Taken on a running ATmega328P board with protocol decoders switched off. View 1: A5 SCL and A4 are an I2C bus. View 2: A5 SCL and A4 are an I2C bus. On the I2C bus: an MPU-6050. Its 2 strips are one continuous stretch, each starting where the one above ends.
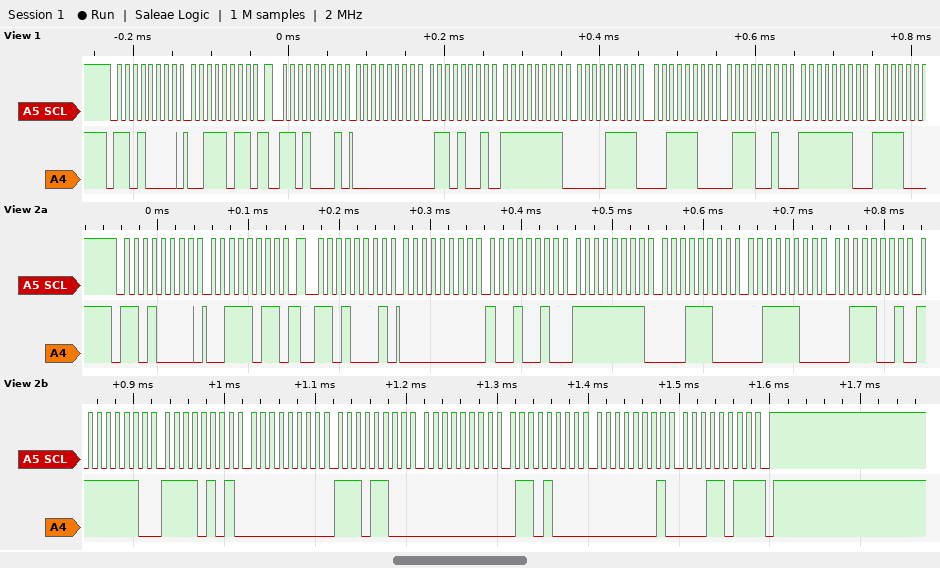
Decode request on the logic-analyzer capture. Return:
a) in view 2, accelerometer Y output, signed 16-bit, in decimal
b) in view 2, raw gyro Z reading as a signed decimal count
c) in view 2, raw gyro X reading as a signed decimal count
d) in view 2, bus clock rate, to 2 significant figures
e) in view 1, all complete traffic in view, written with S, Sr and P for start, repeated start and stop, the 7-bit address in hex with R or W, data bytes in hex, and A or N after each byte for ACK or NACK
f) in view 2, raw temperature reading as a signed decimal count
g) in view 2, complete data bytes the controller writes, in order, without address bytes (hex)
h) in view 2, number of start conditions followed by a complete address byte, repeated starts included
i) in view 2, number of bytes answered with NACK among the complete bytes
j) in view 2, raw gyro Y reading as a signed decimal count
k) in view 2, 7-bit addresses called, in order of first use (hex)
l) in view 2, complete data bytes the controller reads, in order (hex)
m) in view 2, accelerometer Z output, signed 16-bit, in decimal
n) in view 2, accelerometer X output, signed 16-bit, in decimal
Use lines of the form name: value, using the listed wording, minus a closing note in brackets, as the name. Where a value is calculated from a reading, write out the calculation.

in view 2, accelerometer Y output, signed 16-bit, in decimal: 0xFF1C = -228
in view 2, raw gyro Z reading as a signed decimal count: 0x011B = 283
in view 2, raw gyro X reading as a signed decimal count: 0x00EC = 236
in view 2, bus clock rate, to 2 significant figures: 100 kHz
in view 1, all complete traffic in view, written with S, Sr and P for start, repeated start and stop, the 7-bit address in hex with R or W, data bytes in hex, and A or N after each byte for ACK or NACK: S 68W A 3B A Sr 68R A 00 A 69 A FF A 0F A 3C A 72 A FE A
in view 2, raw temperature reading as a signed decimal count: 0xFEF5 = -267
in view 2, complete data bytes the controller writes, in order, without address bytes: 3B
in view 2, number of start conditions followed by a complete address byte, repeated starts included: 2
in view 2, number of bytes answered with NACK among the complete bytes: 1
in view 2, raw gyro Y reading as a signed decimal count: 0x0068 = 104
in view 2, 7-bit addresses called, in order of first use: 0x68
in view 2, complete data bytes the controller reads, in order: 00 92 FF 1C 3C 39 FE F5 00 EC 00 68 01 1B
in view 2, accelerometer Z output, signed 16-bit, in decimal: 0x3C39 = 15417
in view 2, accelerometer X output, signed 16-bit, in decimal: 0x0092 = 146
